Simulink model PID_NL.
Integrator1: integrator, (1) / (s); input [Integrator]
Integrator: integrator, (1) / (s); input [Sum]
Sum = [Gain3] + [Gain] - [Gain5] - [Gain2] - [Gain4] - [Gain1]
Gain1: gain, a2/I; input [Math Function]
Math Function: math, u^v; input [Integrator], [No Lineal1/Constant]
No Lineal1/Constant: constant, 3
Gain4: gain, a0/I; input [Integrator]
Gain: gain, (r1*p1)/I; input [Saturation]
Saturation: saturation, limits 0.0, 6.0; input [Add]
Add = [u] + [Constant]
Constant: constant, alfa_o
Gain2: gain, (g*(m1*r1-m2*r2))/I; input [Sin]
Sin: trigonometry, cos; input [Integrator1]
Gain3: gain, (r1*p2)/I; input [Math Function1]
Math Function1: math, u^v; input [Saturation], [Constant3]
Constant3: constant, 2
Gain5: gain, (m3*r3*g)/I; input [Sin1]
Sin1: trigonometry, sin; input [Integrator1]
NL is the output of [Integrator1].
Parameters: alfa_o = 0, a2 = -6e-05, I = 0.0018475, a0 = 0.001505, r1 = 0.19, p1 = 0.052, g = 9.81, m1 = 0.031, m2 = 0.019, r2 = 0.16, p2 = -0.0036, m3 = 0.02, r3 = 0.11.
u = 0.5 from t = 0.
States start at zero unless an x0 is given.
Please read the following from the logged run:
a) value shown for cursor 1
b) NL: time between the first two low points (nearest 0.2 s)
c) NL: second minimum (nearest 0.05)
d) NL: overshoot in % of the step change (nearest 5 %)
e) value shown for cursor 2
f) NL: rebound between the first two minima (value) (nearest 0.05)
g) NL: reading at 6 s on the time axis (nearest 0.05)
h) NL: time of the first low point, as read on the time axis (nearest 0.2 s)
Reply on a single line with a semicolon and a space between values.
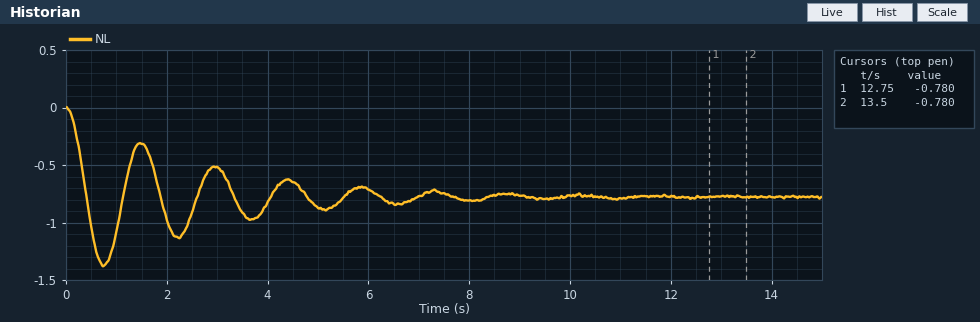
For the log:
-0.780; 1.4 s; -1.15; 75 %; -0.780; -0.30; -0.70; 0.8 s
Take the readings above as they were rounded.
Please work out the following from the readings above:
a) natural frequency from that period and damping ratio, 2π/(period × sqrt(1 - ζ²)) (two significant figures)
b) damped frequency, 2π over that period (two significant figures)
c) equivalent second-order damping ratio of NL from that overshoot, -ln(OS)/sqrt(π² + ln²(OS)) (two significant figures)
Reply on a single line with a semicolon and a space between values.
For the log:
4.5 rad/s; 4.5 rad/s; 0.091
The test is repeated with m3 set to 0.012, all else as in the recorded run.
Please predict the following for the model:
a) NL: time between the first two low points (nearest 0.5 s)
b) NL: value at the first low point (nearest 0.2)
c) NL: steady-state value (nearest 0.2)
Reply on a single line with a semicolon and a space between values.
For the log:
1.5 s; -1.8; -1.0
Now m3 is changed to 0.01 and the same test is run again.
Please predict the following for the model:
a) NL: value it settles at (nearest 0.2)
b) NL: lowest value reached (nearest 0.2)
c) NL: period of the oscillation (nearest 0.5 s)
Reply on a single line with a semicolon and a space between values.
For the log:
-1.0; -1.8; 1.5 s
